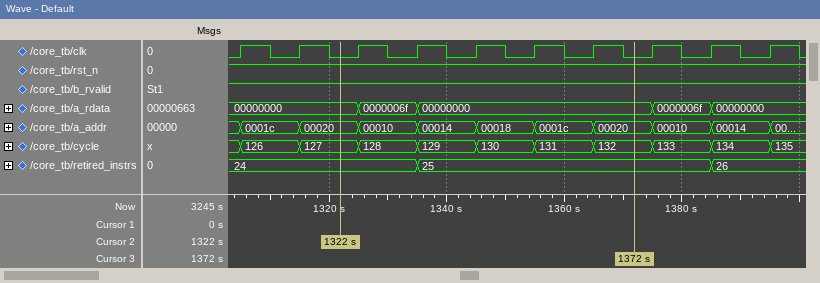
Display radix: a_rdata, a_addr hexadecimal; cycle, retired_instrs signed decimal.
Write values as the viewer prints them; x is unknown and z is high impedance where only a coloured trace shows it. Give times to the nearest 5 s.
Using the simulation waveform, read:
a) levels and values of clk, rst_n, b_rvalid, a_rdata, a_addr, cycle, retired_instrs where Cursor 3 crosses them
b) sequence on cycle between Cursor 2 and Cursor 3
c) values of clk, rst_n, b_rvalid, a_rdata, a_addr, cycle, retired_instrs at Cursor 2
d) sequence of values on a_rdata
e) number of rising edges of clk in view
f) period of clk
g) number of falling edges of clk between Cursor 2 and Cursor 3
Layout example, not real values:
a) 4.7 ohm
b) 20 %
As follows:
a) clk=0, rst_n=1, b_rvalid=1, a_rdata=00000000, a_addr=00020, cycle=132, retired_instrs=25
b) 127, 128, 129, 130, 131, 132
c) clk=0, rst_n=1, b_rvalid=1, a_rdata=00000000, a_addr=00020, cycle=127, retired_instrs=24
d) 00000000, 0000006f, 00000000, 0000006f, 00000000
e) 10
f) 10 s
g) 5
